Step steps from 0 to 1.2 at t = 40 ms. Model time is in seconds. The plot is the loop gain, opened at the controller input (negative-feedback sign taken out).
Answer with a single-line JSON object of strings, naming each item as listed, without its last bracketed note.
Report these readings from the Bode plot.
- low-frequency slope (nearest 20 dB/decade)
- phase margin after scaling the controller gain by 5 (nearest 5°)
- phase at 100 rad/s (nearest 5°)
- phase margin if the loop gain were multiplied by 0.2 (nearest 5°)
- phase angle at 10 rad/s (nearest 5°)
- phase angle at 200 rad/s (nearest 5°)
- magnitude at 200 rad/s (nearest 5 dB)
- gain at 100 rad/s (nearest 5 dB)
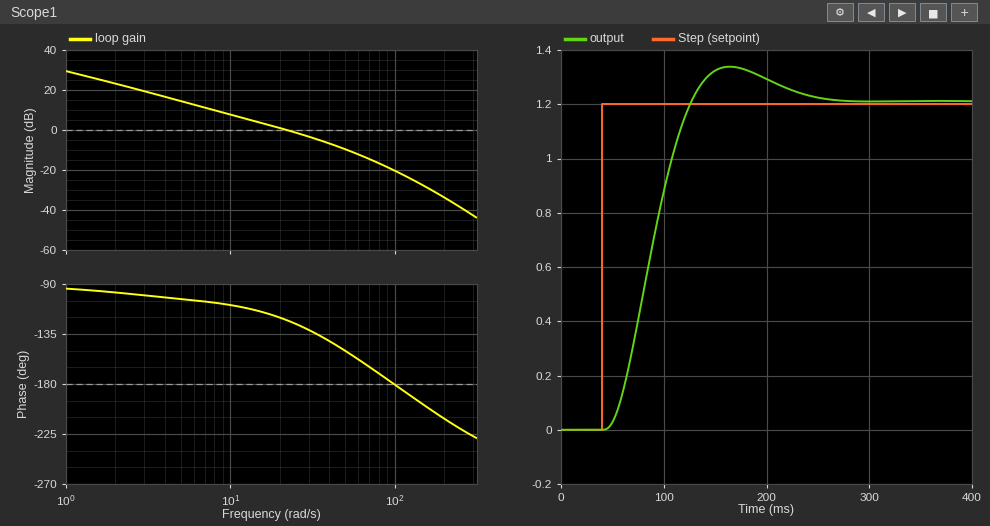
{"low-frequency slope": "-20 dB/decade", "phase margin after scaling the controller gain by 5": "15°", "phase at 100 rad/s": "-180°", "phase margin if the loop gain were multiplied by 0.2": "75°", "phase angle at 10 rad/s": "-110°", "phase angle at 200 rad/s": "-210°", "magnitude at 200 rad/s": "-35 dB", "gain at 100 rad/s": "-20 dB"}
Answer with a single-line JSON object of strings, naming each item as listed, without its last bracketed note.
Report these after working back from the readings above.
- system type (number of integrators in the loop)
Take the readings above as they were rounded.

{"system type": "1"}
